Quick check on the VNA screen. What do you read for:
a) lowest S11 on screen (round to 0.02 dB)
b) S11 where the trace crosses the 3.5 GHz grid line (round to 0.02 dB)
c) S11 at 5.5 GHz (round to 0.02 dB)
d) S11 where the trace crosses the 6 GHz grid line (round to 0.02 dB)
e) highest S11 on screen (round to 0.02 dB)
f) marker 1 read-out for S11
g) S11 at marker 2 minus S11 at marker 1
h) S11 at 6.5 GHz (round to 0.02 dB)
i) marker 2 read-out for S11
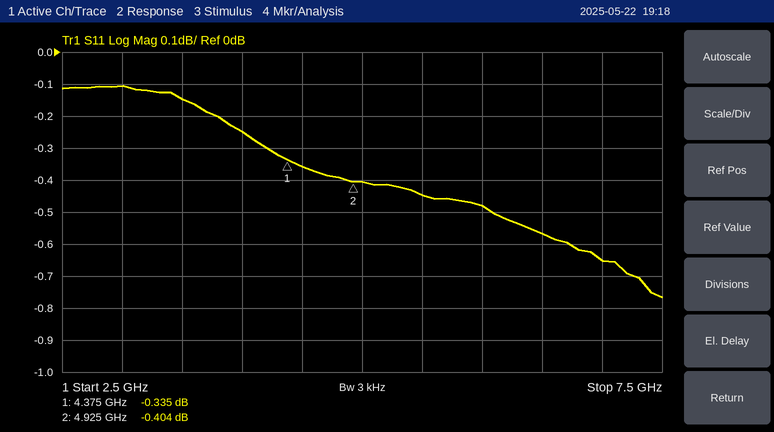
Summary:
-0.76 dB
-0.14 dB
-0.44 dB
-0.48 dB
-0.10 dB
-0.335 dB
-0.069 dB
-0.56 dB
-0.404 dB
